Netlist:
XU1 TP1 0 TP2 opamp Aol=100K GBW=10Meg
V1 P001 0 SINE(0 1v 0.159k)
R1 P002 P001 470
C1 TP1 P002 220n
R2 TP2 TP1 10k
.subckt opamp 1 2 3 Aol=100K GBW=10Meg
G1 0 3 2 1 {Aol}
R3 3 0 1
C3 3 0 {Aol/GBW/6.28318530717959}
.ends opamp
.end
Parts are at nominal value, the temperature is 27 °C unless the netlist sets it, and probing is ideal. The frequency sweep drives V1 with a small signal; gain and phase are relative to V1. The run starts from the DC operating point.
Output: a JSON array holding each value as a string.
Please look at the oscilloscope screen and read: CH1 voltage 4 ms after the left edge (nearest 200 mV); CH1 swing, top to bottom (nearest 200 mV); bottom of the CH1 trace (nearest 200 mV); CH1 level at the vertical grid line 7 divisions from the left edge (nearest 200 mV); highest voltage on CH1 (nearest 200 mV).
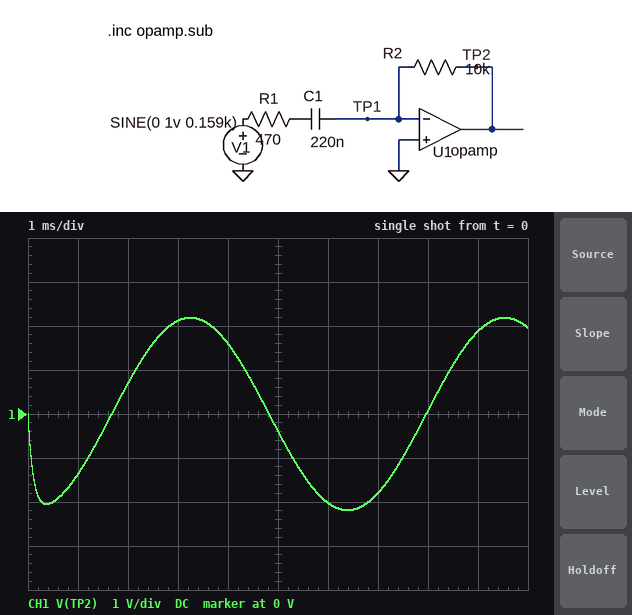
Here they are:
["1.6 V", "4.4 V", "-2.2 V", "-1.8 V", "2.2 V"]
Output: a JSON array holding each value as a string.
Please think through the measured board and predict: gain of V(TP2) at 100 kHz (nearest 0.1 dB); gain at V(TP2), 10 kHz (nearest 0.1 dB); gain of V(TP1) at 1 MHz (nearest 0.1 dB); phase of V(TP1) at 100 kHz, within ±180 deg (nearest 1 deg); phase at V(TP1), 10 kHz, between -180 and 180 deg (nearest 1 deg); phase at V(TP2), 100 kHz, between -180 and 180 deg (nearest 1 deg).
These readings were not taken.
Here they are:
["26.4 dB", "26.5 dB", "-1.2 dB", "78 deg", "97 deg", "168 deg"]
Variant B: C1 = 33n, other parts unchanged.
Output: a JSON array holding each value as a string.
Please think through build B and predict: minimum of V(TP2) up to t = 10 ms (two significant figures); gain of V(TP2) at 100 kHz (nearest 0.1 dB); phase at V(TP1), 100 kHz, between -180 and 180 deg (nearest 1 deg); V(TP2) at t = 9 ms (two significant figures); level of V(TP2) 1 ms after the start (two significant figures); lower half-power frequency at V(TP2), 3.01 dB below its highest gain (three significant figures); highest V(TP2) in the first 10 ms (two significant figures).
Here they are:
["-330 mV", "26.5 dB", "83 deg", "300 mV", "-180 mV", "10.0 kHz", "330 mV"]
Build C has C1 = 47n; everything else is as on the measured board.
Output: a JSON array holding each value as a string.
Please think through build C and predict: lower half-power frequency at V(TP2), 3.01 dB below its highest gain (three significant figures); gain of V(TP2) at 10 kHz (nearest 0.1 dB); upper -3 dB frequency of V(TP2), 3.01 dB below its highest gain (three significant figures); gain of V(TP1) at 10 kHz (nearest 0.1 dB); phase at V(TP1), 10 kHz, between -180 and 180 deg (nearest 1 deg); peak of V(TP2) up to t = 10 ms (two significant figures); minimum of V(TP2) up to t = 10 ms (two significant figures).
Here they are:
["7.09 kHz", "24.8 dB", "456 kHz", "-35.2 dB", "124 deg", "470 mV", "-470 mV"]
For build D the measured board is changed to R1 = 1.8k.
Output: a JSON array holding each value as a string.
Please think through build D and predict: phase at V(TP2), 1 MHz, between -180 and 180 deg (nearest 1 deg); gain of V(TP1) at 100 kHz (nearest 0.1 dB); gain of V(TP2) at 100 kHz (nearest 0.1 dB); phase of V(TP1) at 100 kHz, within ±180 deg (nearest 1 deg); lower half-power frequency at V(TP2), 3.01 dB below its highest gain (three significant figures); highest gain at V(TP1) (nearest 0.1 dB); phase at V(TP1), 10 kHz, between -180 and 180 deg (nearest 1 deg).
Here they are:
["147 deg", "-25.1 dB", "14.9 dB", "86 deg", "402 Hz", "-1.4 dB", "91 deg"]
